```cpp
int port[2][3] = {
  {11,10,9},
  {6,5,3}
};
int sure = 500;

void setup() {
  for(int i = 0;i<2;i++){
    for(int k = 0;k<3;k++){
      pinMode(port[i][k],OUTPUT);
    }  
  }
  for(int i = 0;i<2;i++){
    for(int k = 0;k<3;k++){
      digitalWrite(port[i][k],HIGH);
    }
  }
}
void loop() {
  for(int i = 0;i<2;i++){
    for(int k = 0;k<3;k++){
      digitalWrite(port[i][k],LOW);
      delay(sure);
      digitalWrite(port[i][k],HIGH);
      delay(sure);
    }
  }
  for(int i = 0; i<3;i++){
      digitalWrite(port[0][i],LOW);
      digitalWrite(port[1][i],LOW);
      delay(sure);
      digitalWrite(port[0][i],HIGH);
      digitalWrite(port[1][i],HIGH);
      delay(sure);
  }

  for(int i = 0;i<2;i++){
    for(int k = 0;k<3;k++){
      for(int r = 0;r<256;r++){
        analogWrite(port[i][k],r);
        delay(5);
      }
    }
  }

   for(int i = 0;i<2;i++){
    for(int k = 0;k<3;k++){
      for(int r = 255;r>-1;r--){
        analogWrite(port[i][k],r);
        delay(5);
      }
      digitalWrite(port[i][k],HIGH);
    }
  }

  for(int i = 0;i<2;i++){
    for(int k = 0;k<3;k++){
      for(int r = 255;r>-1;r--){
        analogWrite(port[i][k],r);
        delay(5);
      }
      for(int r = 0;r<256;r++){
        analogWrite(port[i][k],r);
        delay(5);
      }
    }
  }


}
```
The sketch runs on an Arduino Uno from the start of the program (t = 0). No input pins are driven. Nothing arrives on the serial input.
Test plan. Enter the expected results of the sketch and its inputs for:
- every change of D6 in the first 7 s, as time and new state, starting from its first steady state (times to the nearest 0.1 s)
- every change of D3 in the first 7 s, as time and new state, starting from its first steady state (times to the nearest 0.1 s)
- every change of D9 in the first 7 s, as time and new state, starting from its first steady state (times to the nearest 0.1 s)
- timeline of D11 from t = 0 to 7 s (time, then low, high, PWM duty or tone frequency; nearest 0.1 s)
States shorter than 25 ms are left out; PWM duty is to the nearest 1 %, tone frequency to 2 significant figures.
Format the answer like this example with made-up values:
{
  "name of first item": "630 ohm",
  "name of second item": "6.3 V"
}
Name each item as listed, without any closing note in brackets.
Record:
{
  "every change of D6 in the first 7 s, as time and new state, starting from its first steady state": "0 s high; 3 s low; 3.5 s high; 6 s low; 6.5 s high",
  "every change of D3 in the first 7 s, as time and new state, starting from its first steady state": "0 s high; 5 s low; 5.5 s high",
  "every change of D9 in the first 7 s, as time and new state, starting from its first steady state": "0 s high; 2 s low; 2.5 s high",
  "timeline of D11 from t = 0 to 7 s": "0 s low; 0.5 s high; 6 s low; 6.5 s high"
}
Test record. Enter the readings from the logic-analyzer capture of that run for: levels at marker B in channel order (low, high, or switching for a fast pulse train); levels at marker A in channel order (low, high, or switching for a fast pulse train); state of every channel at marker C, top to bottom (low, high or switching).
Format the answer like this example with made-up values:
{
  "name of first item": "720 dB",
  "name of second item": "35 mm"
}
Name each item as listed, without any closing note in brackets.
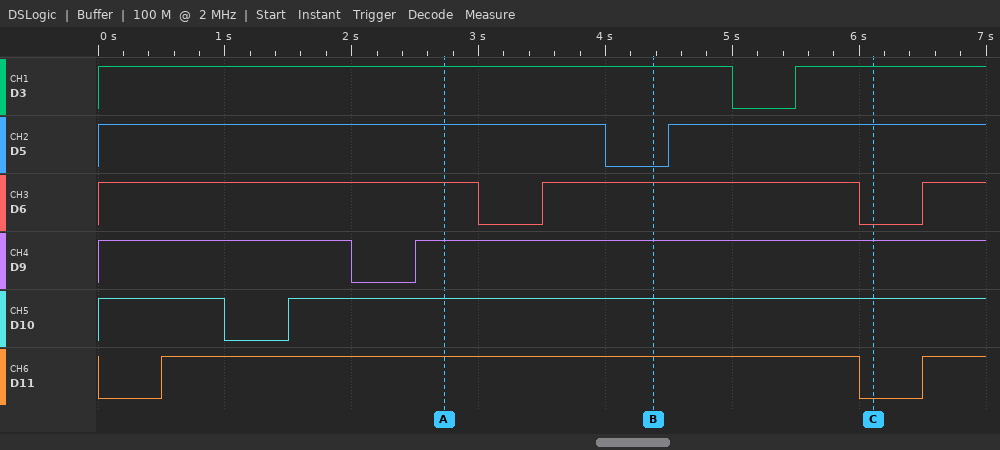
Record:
{
  "levels at marker B in channel order": "D3 high, D5 low, D6 high, D9 high, D10 high, D11 high",
  "levels at marker A in channel order": "D3 high, D5 high, D6 high, D9 high, D10 high, D11 high",
  "state of every channel at marker C, top to bottom": "D3 high, D5 high, D6 low, D9 high, D10 high, D11 low"
}
